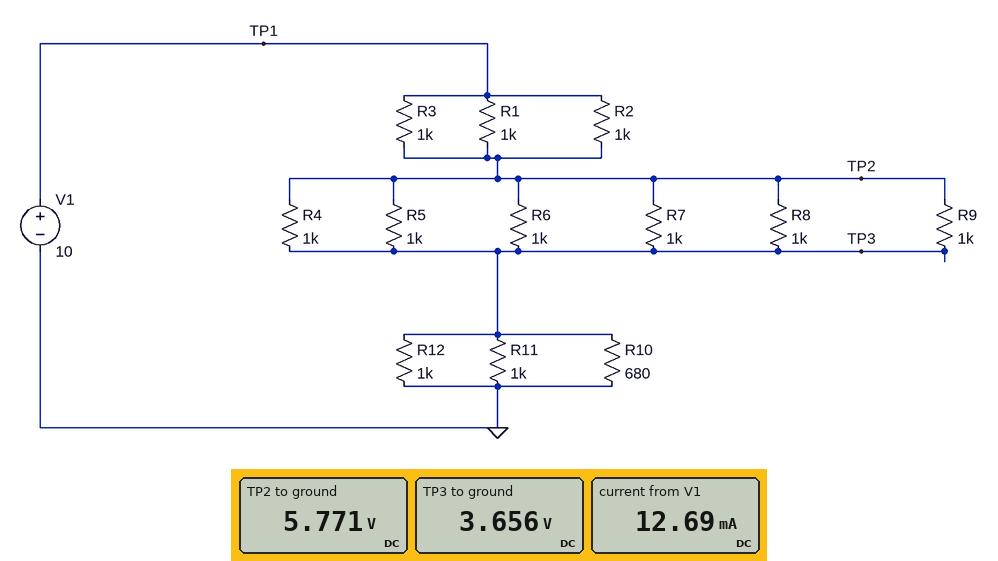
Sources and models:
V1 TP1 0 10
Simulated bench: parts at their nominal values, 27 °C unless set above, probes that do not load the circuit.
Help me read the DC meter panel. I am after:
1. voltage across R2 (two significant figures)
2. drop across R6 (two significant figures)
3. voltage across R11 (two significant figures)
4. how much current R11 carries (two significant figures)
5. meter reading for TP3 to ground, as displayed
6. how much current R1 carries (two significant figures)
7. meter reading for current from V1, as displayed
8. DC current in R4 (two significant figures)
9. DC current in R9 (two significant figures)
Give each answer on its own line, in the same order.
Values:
4.2 V
2.1 V
3.7 V
3.7 mA
3.656 V
4.2 mA
12.69 mA
2.1 mA
2.1 mA
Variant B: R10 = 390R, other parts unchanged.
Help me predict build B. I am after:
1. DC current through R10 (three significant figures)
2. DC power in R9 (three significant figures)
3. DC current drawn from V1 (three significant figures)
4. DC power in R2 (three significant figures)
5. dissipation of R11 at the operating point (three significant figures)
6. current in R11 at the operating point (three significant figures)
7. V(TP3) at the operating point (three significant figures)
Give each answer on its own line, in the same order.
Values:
7.81 mA
5.37 mW
13.9 mA
21.5 mW
9.28 mW
3.05 mA
3.05 V
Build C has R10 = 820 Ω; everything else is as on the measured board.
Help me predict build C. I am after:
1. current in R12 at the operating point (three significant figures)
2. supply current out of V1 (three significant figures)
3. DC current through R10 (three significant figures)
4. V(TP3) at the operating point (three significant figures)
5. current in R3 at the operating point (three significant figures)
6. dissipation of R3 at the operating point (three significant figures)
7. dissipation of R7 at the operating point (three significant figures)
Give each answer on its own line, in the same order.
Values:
3.83 mA
12.3 mA
4.67 mA
3.83 V
4.11 mA
16.9 mW
4.23 mW
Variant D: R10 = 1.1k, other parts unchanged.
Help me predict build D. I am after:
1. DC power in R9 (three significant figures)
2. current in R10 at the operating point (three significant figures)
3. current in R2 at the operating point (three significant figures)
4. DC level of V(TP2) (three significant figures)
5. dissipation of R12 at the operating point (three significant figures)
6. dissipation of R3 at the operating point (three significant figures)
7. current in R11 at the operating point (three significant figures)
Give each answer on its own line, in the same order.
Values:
3.90 mW
3.70 mA
3.95 mA
6.05 V
16.6 mW
15.6 mW
4.07 mA
